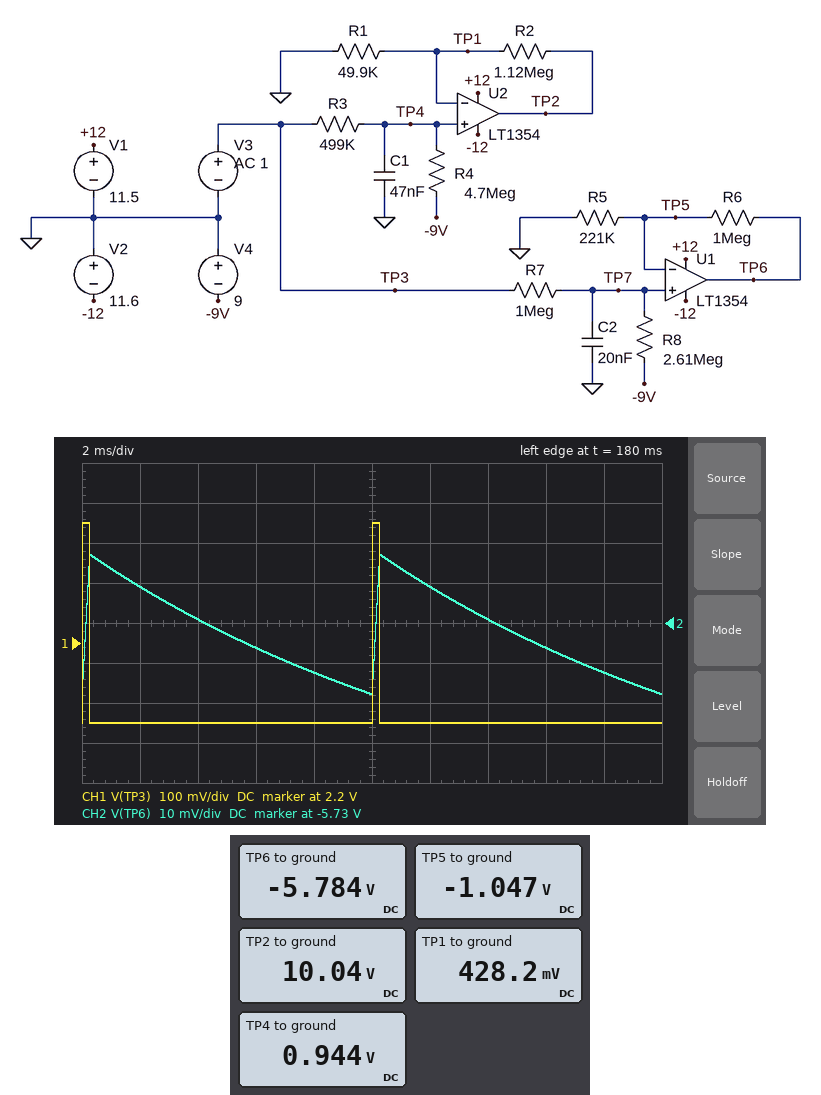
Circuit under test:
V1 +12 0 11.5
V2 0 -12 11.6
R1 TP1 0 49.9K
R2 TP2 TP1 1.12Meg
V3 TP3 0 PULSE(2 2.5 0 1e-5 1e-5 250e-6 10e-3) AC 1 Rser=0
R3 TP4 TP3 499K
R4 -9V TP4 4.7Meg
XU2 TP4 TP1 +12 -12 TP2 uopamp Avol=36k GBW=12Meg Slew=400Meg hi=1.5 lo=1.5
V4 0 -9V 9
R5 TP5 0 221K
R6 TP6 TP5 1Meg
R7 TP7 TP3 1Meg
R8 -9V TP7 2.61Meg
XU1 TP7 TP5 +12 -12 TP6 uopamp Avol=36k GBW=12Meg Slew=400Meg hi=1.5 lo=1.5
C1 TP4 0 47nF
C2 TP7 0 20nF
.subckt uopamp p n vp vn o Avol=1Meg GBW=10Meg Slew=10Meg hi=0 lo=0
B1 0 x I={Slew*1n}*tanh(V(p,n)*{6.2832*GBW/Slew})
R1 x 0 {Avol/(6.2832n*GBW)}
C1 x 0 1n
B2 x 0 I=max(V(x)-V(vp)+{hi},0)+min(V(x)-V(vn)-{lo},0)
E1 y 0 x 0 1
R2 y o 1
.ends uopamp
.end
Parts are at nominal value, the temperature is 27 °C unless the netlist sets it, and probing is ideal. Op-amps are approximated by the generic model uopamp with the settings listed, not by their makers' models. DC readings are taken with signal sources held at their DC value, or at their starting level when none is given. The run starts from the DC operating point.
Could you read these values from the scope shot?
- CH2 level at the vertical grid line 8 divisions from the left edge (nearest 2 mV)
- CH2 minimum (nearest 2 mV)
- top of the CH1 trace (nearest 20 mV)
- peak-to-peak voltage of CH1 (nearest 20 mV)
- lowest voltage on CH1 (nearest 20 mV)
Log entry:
-5.736 V
-5.748 V
2.50 V
500 mV
2.00 V
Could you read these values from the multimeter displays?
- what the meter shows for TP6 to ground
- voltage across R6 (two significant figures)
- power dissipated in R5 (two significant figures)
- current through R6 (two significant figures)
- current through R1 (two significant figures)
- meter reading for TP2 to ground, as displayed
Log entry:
-5.784 V
4.7 V
5.0 µW
4.7 µA
8.6 µA
10.04 V
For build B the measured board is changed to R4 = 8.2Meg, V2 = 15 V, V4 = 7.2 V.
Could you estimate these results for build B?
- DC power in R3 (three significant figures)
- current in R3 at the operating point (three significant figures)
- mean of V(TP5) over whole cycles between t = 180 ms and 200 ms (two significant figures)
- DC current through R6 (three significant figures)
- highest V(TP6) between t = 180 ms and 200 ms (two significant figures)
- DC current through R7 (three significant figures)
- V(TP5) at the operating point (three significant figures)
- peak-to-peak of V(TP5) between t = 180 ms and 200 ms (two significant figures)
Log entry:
558 nW
1.06 µA
-540 mV
2.48 µA
-3.0 V
2.55 µA
-548 mV
6.3 mV
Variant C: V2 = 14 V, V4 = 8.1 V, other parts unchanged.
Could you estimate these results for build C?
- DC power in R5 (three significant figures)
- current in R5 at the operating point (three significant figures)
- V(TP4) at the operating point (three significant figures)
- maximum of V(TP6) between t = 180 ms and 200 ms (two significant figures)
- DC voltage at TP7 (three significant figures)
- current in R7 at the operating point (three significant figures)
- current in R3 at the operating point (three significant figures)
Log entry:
2.88 µW
3.61 µA
1.03 V
-4.3 V
-798 mV
2.80 µA
1.94 µA
